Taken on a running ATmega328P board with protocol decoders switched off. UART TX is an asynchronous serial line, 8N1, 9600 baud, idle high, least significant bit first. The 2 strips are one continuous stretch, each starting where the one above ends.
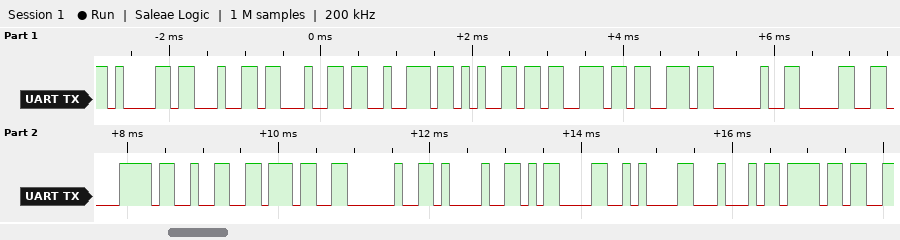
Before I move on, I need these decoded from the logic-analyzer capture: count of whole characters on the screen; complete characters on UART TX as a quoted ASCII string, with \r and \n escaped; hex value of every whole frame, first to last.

18
"address 0x27 !\r\nDo"
61 64 64 72 65 73 73 20 30 78 32 37 20 21 0D 0A 44 6F
